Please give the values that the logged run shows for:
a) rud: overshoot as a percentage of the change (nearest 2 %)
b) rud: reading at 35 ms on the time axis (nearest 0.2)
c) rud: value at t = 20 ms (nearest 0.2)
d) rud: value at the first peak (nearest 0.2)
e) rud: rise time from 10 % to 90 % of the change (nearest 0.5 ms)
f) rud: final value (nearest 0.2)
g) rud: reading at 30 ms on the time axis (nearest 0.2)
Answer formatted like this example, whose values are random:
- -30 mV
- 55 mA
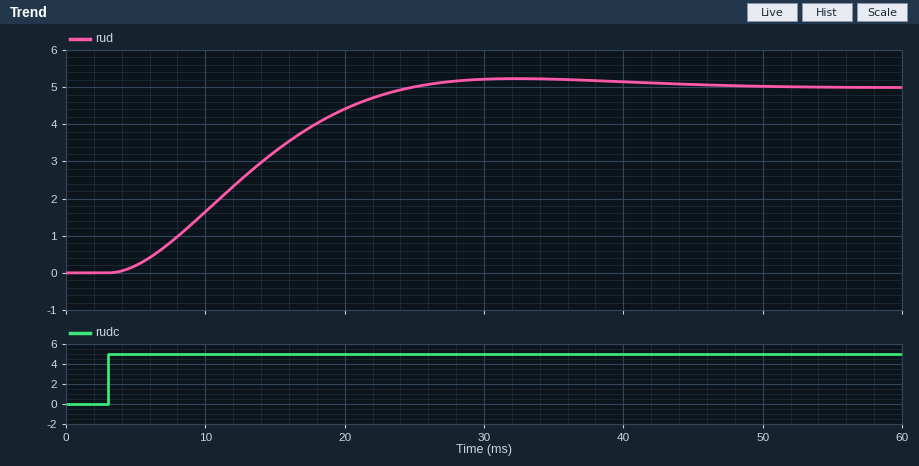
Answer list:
- 4 %
- 5.2
- 4.4
- 5.2
- 14.0 ms
- 5.0
- 5.2
